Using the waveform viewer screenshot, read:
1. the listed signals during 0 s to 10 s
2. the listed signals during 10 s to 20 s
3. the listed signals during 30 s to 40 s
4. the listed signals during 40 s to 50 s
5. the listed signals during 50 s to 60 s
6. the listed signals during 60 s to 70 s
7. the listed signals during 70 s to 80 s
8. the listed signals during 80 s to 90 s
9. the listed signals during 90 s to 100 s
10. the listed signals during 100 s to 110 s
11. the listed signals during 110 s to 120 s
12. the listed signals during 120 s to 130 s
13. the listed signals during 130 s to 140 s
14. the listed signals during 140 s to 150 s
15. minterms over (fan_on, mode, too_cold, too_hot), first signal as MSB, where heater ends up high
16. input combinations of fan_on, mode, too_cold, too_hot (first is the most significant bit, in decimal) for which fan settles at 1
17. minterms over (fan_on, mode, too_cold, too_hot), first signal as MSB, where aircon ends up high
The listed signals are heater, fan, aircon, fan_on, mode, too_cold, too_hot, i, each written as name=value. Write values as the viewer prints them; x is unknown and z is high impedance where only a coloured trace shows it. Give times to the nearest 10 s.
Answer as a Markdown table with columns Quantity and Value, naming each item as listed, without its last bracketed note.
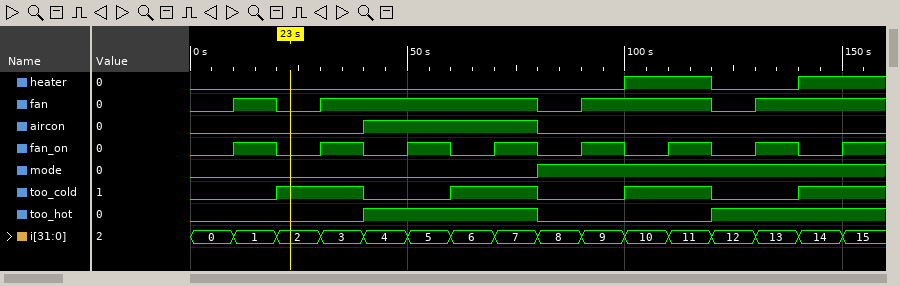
| Quantity | Value |
|---|---|
| the listed signals during 0 s to 10 s | heater=0, fan=0, aircon=0, fan_on=0, mode=0, too_cold=0, too_hot=0, i=0 |
| the listed signals during 10 s to 20 s | heater=0, fan=1, aircon=0, fan_on=1, mode=0, too_cold=0, too_hot=0, i=1 |
| the listed signals during 30 s to 40 s | heater=0, fan=1, aircon=0, fan_on=1, mode=0, too_cold=1, too_hot=0, i=3 |
| the listed signals during 40 s to 50 s | heater=0, fan=1, aircon=1, fan_on=0, mode=0, too_cold=0, too_hot=1, i=4 |
| the listed signals during 50 s to 60 s | heater=0, fan=1, aircon=1, fan_on=1, mode=0, too_cold=0, too_hot=1, i=5 |
| the listed signals during 60 s to 70 s | heater=0, fan=1, aircon=1, fan_on=0, mode=0, too_cold=1, too_hot=1, i=6 |
| the listed signals during 70 s to 80 s | heater=0, fan=1, aircon=1, fan_on=1, mode=0, too_cold=1, too_hot=1, i=7 |
| the listed signals during 80 s to 90 s | heater=0, fan=0, aircon=0, fan_on=0, mode=1, too_cold=0, too_hot=0, i=8 |
| the listed signals during 90 s to 100 s | heater=0, fan=1, aircon=0, fan_on=1, mode=1, too_cold=0, too_hot=0, i=9 |
| the listed signals during 100 s to 110 s | heater=1, fan=1, aircon=0, fan_on=0, mode=1, too_cold=1, too_hot=0, i=10 |
| the listed signals during 110 s to 120 s | heater=1, fan=1, aircon=0, fan_on=1, mode=1, too_cold=1, too_hot=0, i=11 |
| the listed signals during 120 s to 130 s | heater=0, fan=0, aircon=0, fan_on=0, mode=1, too_cold=0, too_hot=1, i=12 |
| the listed signals during 130 s to 140 s | heater=0, fan=1, aircon=0, fan_on=1, mode=1, too_cold=0, too_hot=1, i=13 |
| the listed signals during 140 s to 150 s | heater=1, fan=1, aircon=0, fan_on=0, mode=1, too_cold=1, too_hot=1, i=14 |
| minterms over (fan_on, mode, too_cold, too_hot), first signal as MSB, where heater ends up high | 6, 7, 14, 15 |
| input combinations of fan_on, mode, too_cold, too_hot (first is the most significant bit, in decimal) for which fan settles at 1 | 1, 3, 6, 7, 8, 9, 10, 11, 12, 13, 14, 15 |
| minterms over (fan_on, mode, too_cold, too_hot), first signal as MSB, where aircon ends up high | 1, 3, 9, 11 |
